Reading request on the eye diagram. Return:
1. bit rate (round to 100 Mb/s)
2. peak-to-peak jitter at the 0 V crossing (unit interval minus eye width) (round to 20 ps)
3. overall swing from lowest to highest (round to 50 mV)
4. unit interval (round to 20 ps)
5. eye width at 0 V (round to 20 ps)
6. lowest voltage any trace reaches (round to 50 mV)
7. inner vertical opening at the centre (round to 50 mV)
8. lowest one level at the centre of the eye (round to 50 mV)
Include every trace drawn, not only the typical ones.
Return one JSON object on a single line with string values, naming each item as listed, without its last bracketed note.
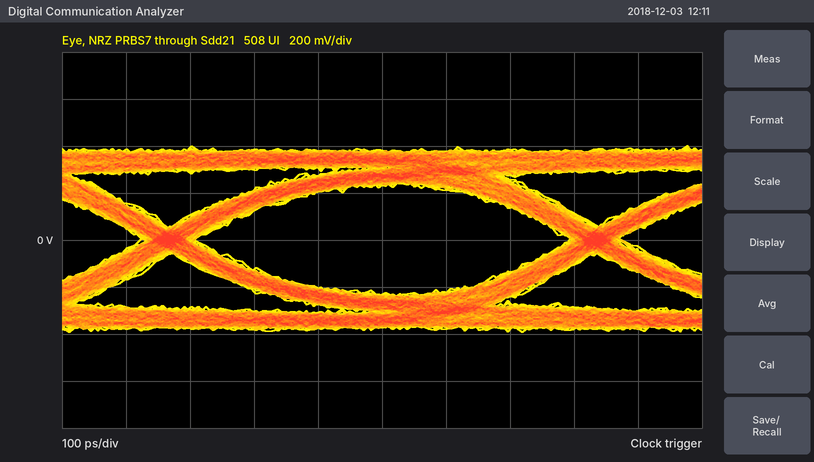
{"bit rate": "1.5 Gb/s", "peak-to-peak jitter at the 0 V crossing (unit interval minus eye width)": "80 ps", "overall swing from lowest to highest": "800 mV", "unit interval": "660 ps", "eye width at 0 V": "580 ps", "lowest voltage any trace reaches": "-400 mV", "inner vertical opening at the centre": "450 mV", "lowest one level at the centre of the eye": "250 mV"}
